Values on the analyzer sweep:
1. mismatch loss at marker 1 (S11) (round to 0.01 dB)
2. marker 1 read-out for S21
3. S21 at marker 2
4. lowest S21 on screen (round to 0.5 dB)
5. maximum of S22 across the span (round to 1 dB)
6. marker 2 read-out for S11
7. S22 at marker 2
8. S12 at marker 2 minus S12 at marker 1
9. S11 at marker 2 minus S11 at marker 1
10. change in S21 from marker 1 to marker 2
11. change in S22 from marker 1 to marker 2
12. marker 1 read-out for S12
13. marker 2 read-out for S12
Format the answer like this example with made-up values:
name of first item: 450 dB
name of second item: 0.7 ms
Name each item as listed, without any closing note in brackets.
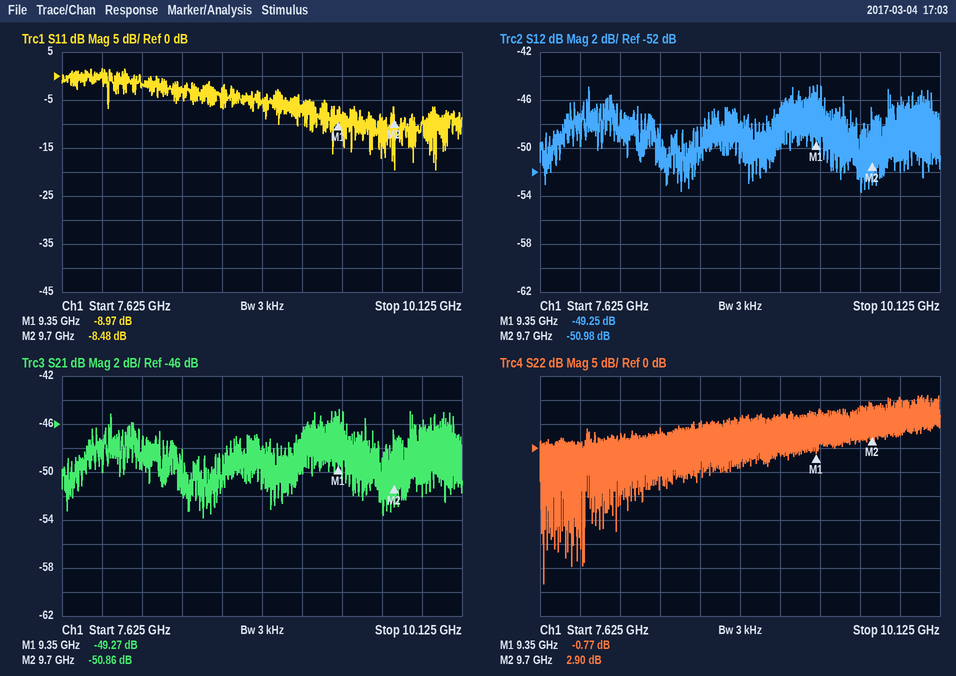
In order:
mismatch loss at marker 1 (S11): 0.59 dB
marker 1 read-out for S21: -49.27 dB
S21 at marker 2: -50.86 dB
lowest S21 on screen: -54.0 dB
maximum of S22 across the span: 11 dB
marker 2 read-out for S11: -8.48 dB
S22 at marker 2: 2.90 dB
S12 at marker 2 minus S12 at marker 1: -1.73 dB
S11 at marker 2 minus S11 at marker 1: 0.49 dB
change in S21 from marker 1 to marker 2: -1.59 dB
change in S22 from marker 1 to marker 2: 3.67 dB
marker 1 read-out for S12: -49.25 dB
marker 2 read-out for S12: -50.98 dB
